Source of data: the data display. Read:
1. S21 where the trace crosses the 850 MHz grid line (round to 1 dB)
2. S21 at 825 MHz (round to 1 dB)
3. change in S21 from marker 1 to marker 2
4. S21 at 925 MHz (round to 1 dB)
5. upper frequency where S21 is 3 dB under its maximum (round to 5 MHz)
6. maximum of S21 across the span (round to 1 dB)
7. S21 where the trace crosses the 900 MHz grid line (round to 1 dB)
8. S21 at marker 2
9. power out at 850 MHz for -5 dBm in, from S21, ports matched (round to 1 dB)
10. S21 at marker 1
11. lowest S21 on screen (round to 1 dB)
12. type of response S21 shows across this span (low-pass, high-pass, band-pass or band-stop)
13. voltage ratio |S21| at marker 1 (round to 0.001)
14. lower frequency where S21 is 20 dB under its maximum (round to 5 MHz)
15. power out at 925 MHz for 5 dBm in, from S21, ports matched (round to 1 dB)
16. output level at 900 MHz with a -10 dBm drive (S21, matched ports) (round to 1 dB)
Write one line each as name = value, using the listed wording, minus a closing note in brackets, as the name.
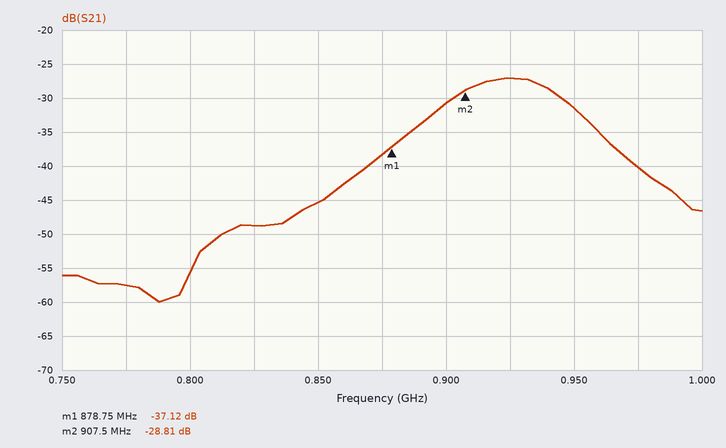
S21 where the trace crosses the 850 MHz grid line = -45 dB
S21 at 825 MHz = -49 dB
change in S21 from marker 1 to marker 2 = 8.31 dB
S21 at 925 MHz = -27 dB
upper frequency where S21 is 3 dB under its maximum = 945 MHz
maximum of S21 across the span = -27 dB
S21 where the trace crosses the 900 MHz grid line = -31 dB
S21 at marker 2 = -28.81 dB
power out at 850 MHz for -5 dBm in, from S21, ports matched = -50 dBm
S21 at marker 1 = -37.12 dB
lowest S21 on screen = -60 dB
type of response S21 shows across this span = band-pass
voltage ratio |S21| at marker 1 = 0.014
lower frequency where S21 is 20 dB under its maximum = 840 MHz
power out at 925 MHz for 5 dBm in, from S21, ports matched = -22 dBm
output level at 900 MHz with a -10 dBm drive (S21, matched ports) = -41 dBm
